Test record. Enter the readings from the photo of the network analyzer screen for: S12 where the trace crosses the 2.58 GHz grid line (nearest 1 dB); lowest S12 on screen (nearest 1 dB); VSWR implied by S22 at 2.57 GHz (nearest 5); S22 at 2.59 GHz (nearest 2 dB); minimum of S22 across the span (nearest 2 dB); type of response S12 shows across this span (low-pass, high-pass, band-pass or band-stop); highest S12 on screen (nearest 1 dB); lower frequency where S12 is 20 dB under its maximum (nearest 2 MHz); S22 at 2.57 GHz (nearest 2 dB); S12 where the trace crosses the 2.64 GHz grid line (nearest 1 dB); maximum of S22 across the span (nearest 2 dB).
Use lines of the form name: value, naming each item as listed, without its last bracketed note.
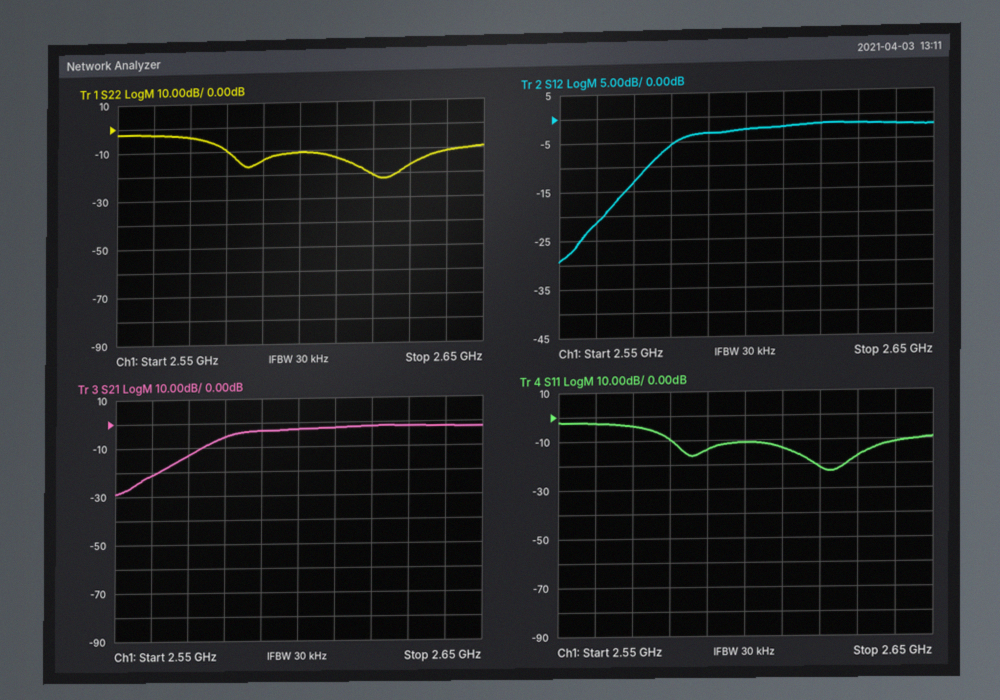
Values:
S12 where the trace crosses the 2.58 GHz grid line: -6 dB
lowest S12 on screen: -29 dB
VSWR implied by S22 at 2.57 GHz: 5
S22 at 2.59 GHz: -14 dB
minimum of S22 across the span: -22 dB
type of response S12 shows across this span: high-pass
highest S12 on screen: -2 dB
lower frequency where S12 is 20 dB under its maximum: 2.560 GHz
S22 at 2.57 GHz: -4 dB
S12 where the trace crosses the 2.64 GHz grid line: -2 dB
maximum of S22 across the span: -2 dB
